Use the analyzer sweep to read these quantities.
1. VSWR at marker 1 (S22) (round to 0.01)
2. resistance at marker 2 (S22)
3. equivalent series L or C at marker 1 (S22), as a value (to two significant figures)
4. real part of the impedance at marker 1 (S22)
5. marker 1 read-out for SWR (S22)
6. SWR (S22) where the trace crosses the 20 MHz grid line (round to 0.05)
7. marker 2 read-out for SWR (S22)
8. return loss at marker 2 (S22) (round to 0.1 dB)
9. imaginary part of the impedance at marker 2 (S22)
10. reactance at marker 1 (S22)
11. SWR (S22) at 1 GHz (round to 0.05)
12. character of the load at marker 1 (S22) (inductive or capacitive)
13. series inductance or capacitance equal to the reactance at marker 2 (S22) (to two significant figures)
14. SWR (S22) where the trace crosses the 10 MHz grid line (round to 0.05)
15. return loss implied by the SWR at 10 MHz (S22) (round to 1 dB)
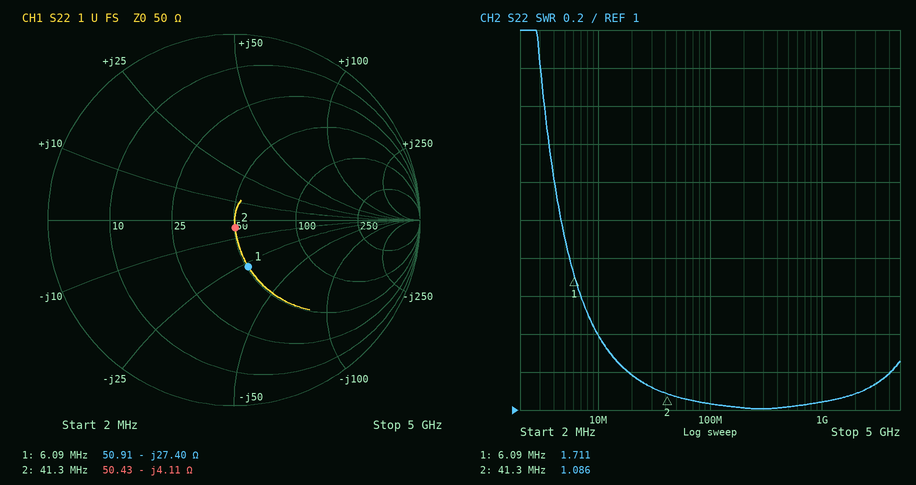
1.71
50.43 Ω
950 pF
50.91 Ω
1.711
1.20
1.086
27.7 dB
-4.11 Ω
-27.40 Ω
1.05
capacitive
940 pF
1.40
16 dB
